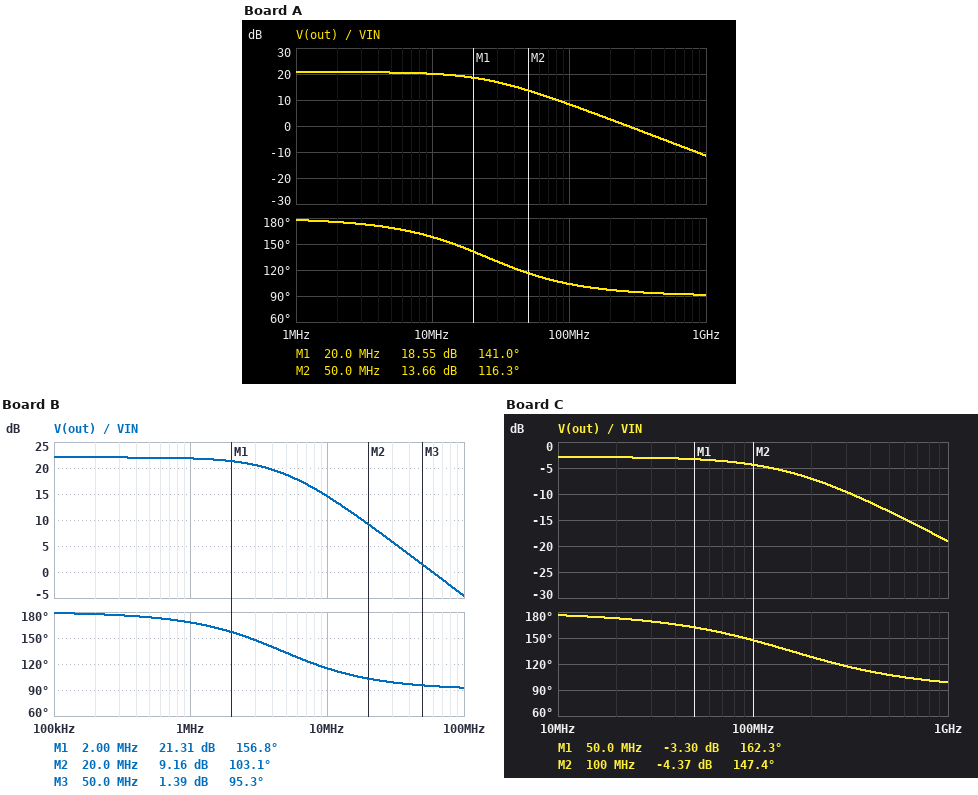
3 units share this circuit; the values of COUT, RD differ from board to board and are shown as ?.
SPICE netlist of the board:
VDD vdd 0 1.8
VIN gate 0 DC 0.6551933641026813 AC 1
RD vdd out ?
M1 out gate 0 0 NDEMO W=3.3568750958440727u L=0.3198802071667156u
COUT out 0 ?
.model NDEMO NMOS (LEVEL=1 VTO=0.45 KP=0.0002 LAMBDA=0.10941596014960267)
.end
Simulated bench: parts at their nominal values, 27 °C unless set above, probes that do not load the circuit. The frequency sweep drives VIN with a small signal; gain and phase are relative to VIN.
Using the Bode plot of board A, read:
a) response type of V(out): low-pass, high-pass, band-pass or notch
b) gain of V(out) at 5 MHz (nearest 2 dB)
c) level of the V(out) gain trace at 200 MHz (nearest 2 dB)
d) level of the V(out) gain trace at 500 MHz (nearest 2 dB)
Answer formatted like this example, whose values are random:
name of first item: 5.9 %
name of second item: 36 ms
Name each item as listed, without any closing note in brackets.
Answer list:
response type of V(out): low-pass, high-pass, band-pass or notch: low-pass
gain of V(out) at 5 MHz: 20 dB
level of the V(out) gain trace at 200 MHz: 2 dB
level of the V(out) gain trace at 500 MHz: -6 dB
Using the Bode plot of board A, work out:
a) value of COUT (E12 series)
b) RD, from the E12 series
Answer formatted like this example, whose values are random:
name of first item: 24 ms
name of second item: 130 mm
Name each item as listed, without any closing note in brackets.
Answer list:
value of COUT: 270 fF
RD, from the E12 series: 27 kΩ
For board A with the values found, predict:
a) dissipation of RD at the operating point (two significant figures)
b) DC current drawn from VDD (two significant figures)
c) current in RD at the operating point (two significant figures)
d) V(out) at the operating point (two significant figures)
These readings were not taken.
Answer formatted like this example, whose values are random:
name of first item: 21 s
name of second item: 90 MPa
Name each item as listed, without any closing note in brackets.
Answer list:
dissipation of RD at the operating point: 59 µW
DC current drawn from VDD: 47 µA
current in RD at the operating point: 47 µA
V(out) at the operating point: 540 mV
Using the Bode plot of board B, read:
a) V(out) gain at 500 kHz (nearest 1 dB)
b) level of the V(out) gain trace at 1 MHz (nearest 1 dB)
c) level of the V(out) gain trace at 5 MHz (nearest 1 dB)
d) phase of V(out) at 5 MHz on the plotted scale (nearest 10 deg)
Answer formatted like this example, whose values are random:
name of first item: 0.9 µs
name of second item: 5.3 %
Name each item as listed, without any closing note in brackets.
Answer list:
V(out) gain at 500 kHz: 22 dB
level of the V(out) gain trace at 1 MHz: 22 dB
level of the V(out) gain trace at 5 MHz: 19 dB
phase of V(out) at 5 MHz on the plotted scale: 130 deg
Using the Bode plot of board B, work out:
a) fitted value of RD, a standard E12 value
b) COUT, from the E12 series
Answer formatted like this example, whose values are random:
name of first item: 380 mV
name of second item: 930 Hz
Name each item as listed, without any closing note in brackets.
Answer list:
fitted value of RD, a standard E12 value: 33 kΩ
COUT, from the E12 series: 1.2 pF
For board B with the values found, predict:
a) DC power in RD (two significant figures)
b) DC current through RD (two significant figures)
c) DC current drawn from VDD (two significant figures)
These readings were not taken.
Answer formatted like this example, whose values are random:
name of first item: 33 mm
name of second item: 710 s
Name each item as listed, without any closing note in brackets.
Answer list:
DC power in RD: 69 µW
DC current through RD: 46 µA
DC current drawn from VDD: 46 µA
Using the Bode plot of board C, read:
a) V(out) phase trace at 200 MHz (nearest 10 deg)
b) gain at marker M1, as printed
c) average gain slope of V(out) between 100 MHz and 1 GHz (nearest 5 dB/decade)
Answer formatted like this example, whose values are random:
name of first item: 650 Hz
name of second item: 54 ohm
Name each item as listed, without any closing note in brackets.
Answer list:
V(out) phase trace at 200 MHz: 130 deg
gain at marker M1, as printed: -3.30 dB
average gain slope of V(out) between 100 MHz and 1 GHz: -15 dB/decade
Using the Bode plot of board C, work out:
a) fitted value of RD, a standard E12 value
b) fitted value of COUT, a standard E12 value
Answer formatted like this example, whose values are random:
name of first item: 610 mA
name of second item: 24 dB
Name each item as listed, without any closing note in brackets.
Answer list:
fitted value of RD, a standard E12 value: 56 kΩ
fitted value of COUT, a standard E12 value: 270 fF
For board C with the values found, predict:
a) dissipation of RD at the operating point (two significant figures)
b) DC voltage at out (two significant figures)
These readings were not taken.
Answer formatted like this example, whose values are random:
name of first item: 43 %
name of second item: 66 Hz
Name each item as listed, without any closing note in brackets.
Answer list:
dissipation of RD at the operating point: 52 µW
DC voltage at out: 90 mV
